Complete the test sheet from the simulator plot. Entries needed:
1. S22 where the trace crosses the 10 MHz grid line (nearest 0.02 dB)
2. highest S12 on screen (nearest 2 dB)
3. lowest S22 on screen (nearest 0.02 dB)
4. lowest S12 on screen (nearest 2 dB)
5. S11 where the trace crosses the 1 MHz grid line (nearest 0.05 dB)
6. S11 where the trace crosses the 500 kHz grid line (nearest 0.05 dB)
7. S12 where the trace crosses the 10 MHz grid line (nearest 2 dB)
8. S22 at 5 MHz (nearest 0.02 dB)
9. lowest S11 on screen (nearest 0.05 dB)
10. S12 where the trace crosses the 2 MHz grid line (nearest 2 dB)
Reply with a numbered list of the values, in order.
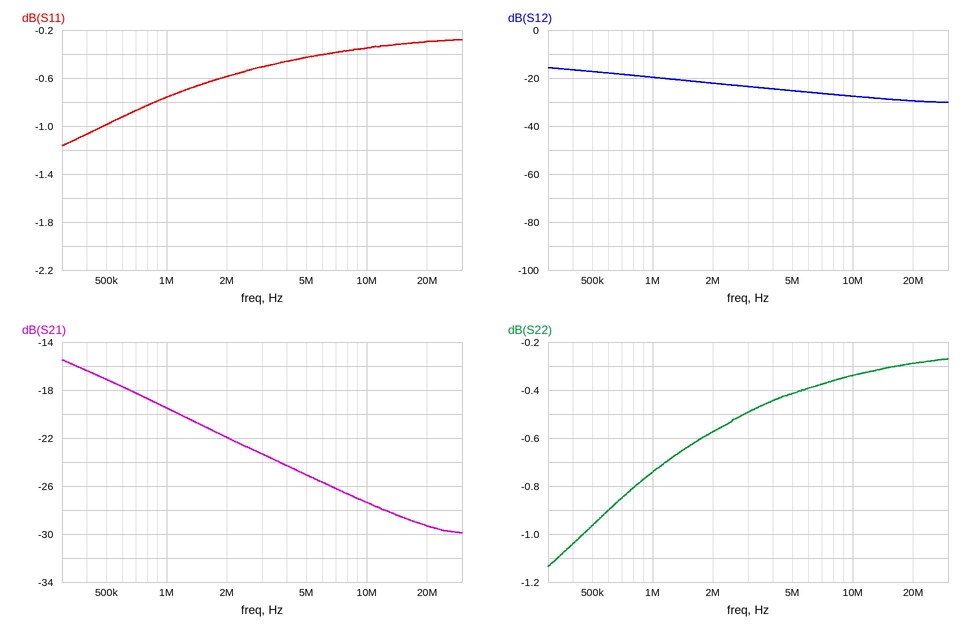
1. -0.34 dB
2. -16 dB
3. -1.14 dB
4. -30 dB
5. -0.75 dB
6. -1.00 dB
7. -28 dB
8. -0.42 dB
9. -1.15 dB
10. -22 dB
